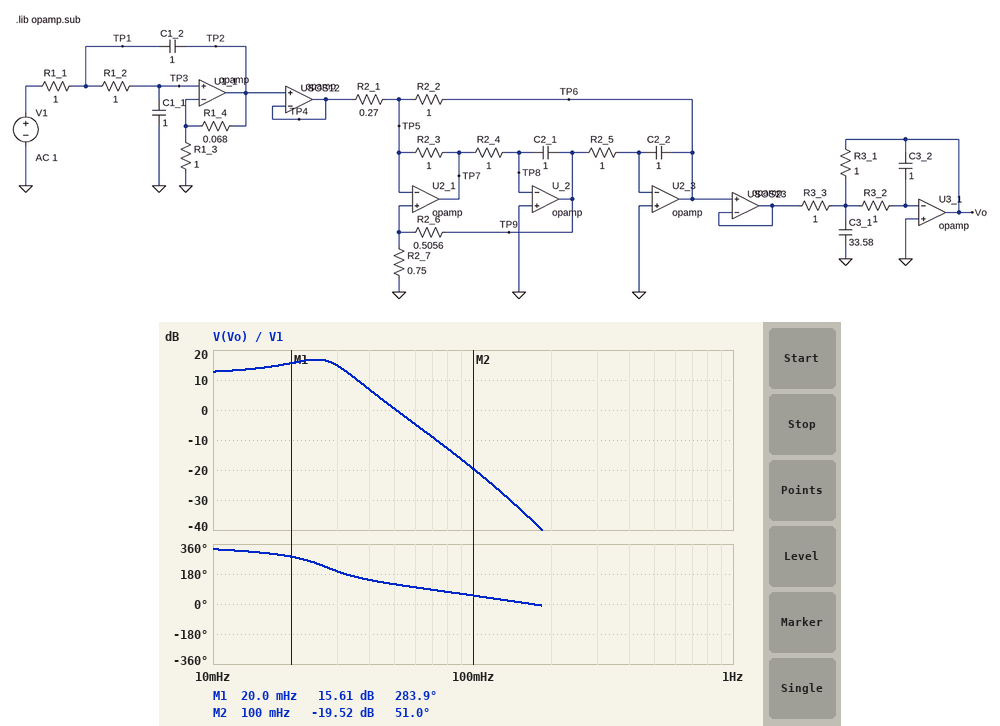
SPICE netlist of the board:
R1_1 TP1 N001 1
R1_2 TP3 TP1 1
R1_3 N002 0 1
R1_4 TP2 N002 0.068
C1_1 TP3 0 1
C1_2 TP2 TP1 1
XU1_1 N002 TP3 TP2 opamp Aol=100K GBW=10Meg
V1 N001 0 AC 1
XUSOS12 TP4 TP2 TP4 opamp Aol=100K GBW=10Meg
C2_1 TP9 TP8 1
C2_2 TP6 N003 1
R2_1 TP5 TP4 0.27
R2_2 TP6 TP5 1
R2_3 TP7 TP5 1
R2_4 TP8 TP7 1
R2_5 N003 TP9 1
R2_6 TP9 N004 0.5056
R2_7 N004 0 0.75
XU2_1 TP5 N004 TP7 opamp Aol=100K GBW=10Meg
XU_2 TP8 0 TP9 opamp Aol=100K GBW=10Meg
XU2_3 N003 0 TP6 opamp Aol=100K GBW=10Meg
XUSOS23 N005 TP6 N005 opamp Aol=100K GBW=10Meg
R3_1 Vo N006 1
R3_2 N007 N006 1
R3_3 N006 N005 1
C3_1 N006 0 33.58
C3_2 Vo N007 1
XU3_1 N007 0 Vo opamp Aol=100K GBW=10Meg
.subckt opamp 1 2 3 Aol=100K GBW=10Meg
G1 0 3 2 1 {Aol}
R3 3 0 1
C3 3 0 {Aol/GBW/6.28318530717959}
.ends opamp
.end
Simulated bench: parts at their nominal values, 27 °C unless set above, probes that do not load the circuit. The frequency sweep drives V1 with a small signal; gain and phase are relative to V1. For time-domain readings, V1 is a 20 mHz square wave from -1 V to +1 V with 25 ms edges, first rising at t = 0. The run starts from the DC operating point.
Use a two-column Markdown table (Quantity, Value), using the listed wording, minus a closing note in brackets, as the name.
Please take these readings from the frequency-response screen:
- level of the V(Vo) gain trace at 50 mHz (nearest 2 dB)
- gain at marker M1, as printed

| Quantity | Value |
|---|---|
| level of the V(Vo) gain trace at 50 mHz | 0 dB |
| gain at marker M1, as printed | 15.61 dB |
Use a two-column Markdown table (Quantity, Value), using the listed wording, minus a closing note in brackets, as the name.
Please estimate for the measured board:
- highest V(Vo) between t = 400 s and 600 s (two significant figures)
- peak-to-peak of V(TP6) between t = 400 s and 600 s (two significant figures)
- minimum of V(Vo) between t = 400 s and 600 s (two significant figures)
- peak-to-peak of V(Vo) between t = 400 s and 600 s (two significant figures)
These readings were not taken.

| Quantity | Value |
|---|---|
| highest V(Vo) between t = 400 s and 600 s | 7.5 V |
| peak-to-peak of V(TP6) between t = 400 s and 600 s | 7.9 V |
| minimum of V(Vo) between t = 400 s and 600 s | -7.5 V |
| peak-to-peak of V(Vo) between t = 400 s and 600 s | 15 V |
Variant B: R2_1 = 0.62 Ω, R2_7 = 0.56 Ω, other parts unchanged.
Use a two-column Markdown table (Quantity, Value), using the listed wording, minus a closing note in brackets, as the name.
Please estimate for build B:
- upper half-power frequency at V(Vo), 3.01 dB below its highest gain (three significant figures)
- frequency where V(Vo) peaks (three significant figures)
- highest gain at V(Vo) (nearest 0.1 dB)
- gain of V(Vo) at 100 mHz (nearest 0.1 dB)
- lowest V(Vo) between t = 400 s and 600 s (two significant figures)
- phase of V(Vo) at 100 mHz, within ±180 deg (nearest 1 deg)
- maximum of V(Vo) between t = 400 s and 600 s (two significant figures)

| Quantity | Value |
|---|---|
| upper half-power frequency at V(Vo), 3.01 dB below its highest gain | 31.8 mHz |
| frequency where V(Vo) peaks | 25.4 mHz |
| highest gain at V(Vo) | 10.4 dB |
| gain of V(Vo) at 100 mHz | -22.3 dB |
| lowest V(Vo) between t = 400 s and 600 s | -3.5 V |
| phase of V(Vo) at 100 mHz, within ±180 deg | 62 deg |
| maximum of V(Vo) between t = 400 s and 600 s | 3.5 V |
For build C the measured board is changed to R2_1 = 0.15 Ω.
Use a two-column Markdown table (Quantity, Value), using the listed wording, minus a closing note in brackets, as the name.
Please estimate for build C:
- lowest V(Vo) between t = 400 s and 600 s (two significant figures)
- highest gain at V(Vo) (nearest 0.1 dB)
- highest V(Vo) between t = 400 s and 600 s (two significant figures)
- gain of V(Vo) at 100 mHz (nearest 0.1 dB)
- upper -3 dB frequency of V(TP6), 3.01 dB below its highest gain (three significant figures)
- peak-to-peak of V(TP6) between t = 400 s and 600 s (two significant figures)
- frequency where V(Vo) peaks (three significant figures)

| Quantity | Value |
|---|---|
| lowest V(Vo) between t = 400 s and 600 s | -12 V |
| highest gain at V(Vo) | 20.8 dB |
| highest V(Vo) between t = 400 s and 600 s | 12 V |
| gain of V(Vo) at 100 mHz | -17.9 dB |
| upper -3 dB frequency of V(TP6), 3.01 dB below its highest gain | 30.0 mHz |
| peak-to-peak of V(TP6) between t = 400 s and 600 s | 14 V |
| frequency where V(Vo) peaks | 24.6 mHz |
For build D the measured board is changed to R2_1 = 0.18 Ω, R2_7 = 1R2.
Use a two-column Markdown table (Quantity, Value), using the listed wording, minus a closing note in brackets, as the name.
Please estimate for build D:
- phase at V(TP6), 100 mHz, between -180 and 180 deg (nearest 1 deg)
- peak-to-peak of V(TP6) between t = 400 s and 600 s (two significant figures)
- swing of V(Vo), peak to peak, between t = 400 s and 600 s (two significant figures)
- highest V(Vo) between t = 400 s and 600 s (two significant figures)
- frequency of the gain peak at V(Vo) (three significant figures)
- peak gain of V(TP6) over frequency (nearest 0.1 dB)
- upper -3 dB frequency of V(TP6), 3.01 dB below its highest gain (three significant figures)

| Quantity | Value |
|---|---|
| phase at V(TP6), 100 mHz, between -180 and 180 deg | 37 deg |
| peak-to-peak of V(TP6) between t = 400 s and 600 s | 12 V |
| swing of V(Vo), peak to peak, between t = 400 s and 600 s | 20 V |
| highest V(Vo) between t = 400 s and 600 s | 10 V |
| frequency of the gain peak at V(Vo) | 24.5 mHz |
| peak gain of V(TP6) over frequency | 15.5 dB |
| upper -3 dB frequency of V(TP6), 3.01 dB below its highest gain | 29.2 mHz |
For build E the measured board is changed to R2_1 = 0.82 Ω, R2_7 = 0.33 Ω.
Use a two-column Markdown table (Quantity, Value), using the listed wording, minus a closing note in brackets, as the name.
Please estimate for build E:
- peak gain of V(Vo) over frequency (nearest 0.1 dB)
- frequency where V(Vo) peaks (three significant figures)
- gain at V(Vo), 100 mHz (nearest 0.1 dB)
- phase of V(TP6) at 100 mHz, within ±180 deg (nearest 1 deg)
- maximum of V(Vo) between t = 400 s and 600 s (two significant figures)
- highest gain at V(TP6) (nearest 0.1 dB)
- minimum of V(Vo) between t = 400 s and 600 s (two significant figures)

| Quantity | Value |
|---|---|
| peak gain of V(Vo) over frequency | 8.2 dB |
| frequency where V(Vo) peaks | 25.5 mHz |
| gain at V(Vo), 100 mHz | -22.2 dB |
| phase of V(TP6) at 100 mHz, within ±180 deg | 64 deg |
| maximum of V(Vo) between t = 400 s and 600 s | 2.7 V |
| highest gain at V(TP6) | 2.3 dB |
| minimum of V(Vo) between t = 400 s and 600 s | -2.7 V |
